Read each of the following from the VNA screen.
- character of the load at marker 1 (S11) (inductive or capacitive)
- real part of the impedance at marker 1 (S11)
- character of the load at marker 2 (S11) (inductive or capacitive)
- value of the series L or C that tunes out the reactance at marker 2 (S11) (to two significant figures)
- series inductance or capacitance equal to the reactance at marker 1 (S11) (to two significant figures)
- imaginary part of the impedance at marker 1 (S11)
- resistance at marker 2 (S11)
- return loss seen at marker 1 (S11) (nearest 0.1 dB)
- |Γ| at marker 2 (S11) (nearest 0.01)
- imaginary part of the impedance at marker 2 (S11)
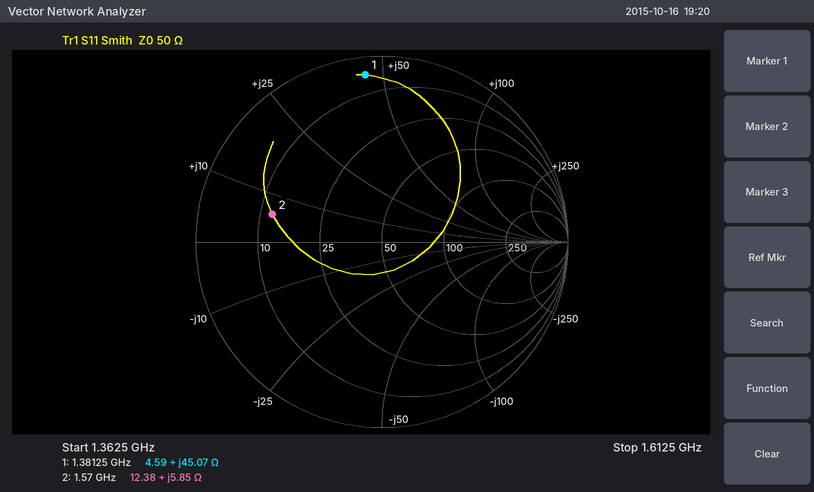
inductive
4.59 Ω
inductive
17 pF
5.2 nH
+45.07 Ω
12.38 Ω
0.9 dB
0.61
+5.85 Ω
